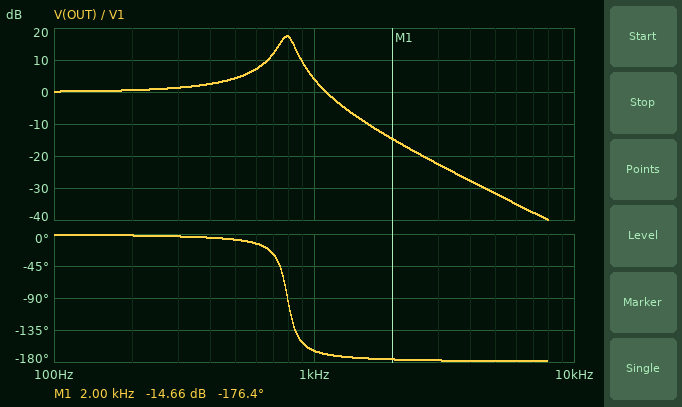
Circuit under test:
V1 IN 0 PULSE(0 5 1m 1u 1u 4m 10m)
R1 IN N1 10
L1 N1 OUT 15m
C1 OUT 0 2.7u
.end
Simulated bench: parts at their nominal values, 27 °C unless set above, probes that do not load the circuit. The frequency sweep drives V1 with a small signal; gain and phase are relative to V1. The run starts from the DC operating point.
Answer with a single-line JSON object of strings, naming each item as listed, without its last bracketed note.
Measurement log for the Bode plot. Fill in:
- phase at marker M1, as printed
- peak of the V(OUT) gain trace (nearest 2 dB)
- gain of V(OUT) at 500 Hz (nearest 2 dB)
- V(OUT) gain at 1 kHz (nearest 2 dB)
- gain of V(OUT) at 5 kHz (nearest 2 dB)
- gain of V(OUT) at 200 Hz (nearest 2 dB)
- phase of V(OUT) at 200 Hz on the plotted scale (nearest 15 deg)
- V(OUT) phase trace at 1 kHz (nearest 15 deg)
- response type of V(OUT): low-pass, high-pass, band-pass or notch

{"phase at marker M1, as printed": "-176.4 deg", "peak of the V(OUT) gain trace": "18 dB", "gain of V(OUT) at 500 Hz": "4 dB", "V(OUT) gain at 1 kHz": "4 dB", "gain of V(OUT) at 5 kHz": "-32 dB", "gain of V(OUT) at 200 Hz": "0 dB", "phase of V(OUT) at 200 Hz on the plotted scale": "0 deg", "V(OUT) phase trace at 1 kHz": "-165 deg", "response type of V(OUT): low-pass, high-pass, band-pass or notch": "low-pass"}
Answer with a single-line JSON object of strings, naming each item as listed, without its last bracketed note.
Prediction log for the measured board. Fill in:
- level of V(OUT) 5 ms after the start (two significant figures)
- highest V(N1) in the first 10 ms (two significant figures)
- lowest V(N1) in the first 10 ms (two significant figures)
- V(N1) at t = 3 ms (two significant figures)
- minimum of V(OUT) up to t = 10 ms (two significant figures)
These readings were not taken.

{"level of V(OUT) 5 ms after the start": "4.2 V", "highest V(N1) in the first 10 ms": "5.5 V", "lowest V(N1) in the first 10 ms": "-430 mV", "V(N1) at t = 3 ms": "5.2 V", "minimum of V(OUT) up to t = 10 ms": "-3.5 V"}
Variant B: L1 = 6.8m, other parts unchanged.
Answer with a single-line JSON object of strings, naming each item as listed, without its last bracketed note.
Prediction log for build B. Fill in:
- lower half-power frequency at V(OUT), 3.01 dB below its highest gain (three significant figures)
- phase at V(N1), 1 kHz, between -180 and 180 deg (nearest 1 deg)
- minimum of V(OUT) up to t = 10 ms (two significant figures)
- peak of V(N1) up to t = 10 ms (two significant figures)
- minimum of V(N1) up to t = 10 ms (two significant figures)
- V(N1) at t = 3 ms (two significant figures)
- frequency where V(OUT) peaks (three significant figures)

{"lower half-power frequency at V(OUT), 3.01 dB below its highest gain": "1.04 kHz", "phase at V(N1), 1 kHz, between -180 and 180 deg": "-32 deg", "minimum of V(OUT) up to t = 10 ms": "-3.8 V", "peak of V(N1) up to t = 10 ms": "5.6 V", "minimum of V(N1) up to t = 10 ms": "-650 mV", "V(N1) at t = 3 ms": "4.8 V", "frequency where V(OUT) peaks": "1.16 kHz"}
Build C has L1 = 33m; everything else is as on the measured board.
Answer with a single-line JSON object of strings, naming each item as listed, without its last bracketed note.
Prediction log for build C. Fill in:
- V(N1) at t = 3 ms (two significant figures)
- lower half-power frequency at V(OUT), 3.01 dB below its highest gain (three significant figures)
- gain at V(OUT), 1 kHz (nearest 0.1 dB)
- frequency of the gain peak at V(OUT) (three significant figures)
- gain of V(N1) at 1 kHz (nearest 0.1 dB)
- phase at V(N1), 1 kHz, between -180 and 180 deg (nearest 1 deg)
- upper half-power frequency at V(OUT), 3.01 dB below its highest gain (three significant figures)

{"V(N1) at t = 3 ms": "4.9 V", "lower half-power frequency at V(OUT), 3.01 dB below its highest gain": "507 Hz", "gain at V(OUT), 1 kHz": "-8.0 dB", "frequency of the gain peak at V(OUT)": "532 Hz", "gain of V(N1) at 1 kHz": "0 dB", "phase at V(N1), 1 kHz, between -180 and 180 deg": "4 deg", "upper half-power frequency at V(OUT), 3.01 dB below its highest gain": "556 Hz"}
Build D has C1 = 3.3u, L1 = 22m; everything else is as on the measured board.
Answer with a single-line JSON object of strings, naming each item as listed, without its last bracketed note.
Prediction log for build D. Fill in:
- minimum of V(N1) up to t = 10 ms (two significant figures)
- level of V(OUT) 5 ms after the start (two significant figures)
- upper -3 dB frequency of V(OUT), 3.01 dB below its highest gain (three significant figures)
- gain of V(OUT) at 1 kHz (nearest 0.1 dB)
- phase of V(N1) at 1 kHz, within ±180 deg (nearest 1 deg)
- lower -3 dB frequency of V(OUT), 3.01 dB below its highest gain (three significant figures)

{"minimum of V(N1) up to t = 10 ms": "-590 mV", "level of V(OUT) 5 ms after the start": "6.2 V", "upper -3 dB frequency of V(OUT), 3.01 dB below its highest gain": "624 Hz", "gain of V(OUT) at 1 kHz": "-5.5 dB", "phase of V(N1) at 1 kHz, within ±180 deg": "6 deg", "lower -3 dB frequency of V(OUT), 3.01 dB below its highest gain": "551 Hz"}
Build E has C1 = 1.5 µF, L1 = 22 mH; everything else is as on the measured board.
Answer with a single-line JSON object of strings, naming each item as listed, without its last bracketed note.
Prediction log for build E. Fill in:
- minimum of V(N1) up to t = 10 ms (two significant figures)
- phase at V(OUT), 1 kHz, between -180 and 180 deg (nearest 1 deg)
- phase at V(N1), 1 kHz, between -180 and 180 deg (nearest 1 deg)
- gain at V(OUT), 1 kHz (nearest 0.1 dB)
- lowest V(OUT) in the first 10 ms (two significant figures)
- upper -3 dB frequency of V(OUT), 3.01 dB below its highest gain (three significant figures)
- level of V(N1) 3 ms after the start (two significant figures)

{"minimum of V(N1) up to t = 10 ms": "-480 mV", "phase at V(OUT), 1 kHz, between -180 and 180 deg": "-163 deg", "phase at V(N1), 1 kHz, between -180 and 180 deg": "17 deg", "gain at V(OUT), 1 kHz": "10.0 dB", "lowest V(OUT) in the first 10 ms": "-6.2 V", "upper -3 dB frequency of V(OUT), 3.01 dB below its highest gain": "910 Hz", "level of V(N1) 3 ms after the start": "5.3 V"}
